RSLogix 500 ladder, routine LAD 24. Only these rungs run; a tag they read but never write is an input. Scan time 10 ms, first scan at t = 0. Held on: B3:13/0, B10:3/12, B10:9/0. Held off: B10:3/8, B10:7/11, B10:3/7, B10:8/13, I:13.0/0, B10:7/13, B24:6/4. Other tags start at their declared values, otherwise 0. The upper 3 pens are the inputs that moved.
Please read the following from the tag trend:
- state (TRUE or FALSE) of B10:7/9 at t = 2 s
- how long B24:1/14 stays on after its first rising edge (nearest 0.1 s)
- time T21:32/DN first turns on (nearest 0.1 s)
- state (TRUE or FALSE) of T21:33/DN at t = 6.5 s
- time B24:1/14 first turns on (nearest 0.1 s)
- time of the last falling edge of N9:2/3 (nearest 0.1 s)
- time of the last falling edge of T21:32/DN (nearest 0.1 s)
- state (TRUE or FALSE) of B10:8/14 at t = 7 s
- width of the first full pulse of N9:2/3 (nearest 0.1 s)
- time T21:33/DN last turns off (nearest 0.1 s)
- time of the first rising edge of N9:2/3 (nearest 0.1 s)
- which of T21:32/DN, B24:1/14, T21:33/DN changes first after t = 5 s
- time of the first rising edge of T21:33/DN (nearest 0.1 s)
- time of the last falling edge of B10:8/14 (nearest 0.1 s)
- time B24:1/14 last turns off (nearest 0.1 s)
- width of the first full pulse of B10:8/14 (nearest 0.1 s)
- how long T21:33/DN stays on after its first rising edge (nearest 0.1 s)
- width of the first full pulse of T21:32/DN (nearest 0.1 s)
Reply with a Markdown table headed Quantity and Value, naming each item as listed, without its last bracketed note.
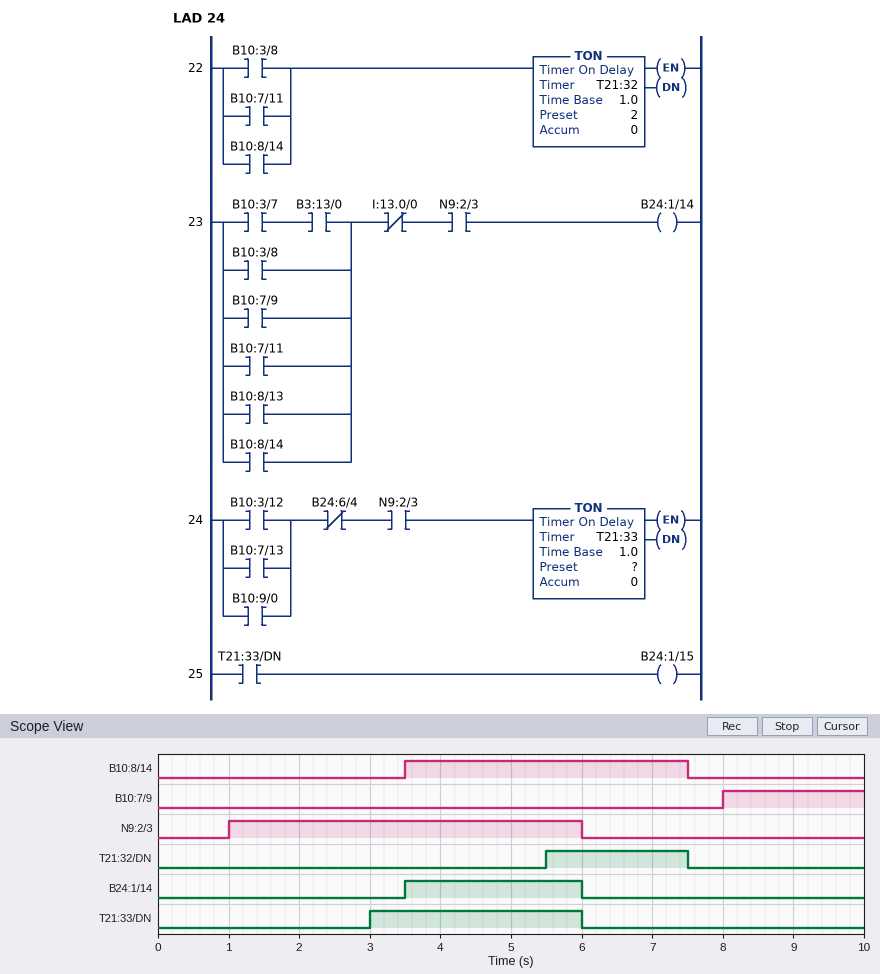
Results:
| Quantity | Value |
|---|---|
| state (TRUE or FALSE) of B10:7/9 at t = 2 s | FALSE |
| how long B24:1/14 stays on after its first rising edge | 2.5 s |
| time T21:32/DN first turns on | 5.5 s |
| state (TRUE or FALSE) of T21:33/DN at t = 6.5 s | FALSE |
| time B24:1/14 first turns on | 3.5 s |
| time of the last falling edge of N9:2/3 | 6.0 s |
| time of the last falling edge of T21:32/DN | 7.5 s |
| state (TRUE or FALSE) of B10:8/14 at t = 7 s | TRUE |
| width of the first full pulse of N9:2/3 | 5.0 s |
| time T21:33/DN last turns off | 6.0 s |
| time of the first rising edge of N9:2/3 | 1.0 s |
| which of T21:32/DN, B24:1/14, T21:33/DN changes first after t = 5 s | T21:32/DN |
| time of the first rising edge of T21:33/DN | 3.0 s |
| time of the last falling edge of B10:8/14 | 7.5 s |
| time B24:1/14 last turns off | 6.0 s |
| width of the first full pulse of B10:8/14 | 4.0 s |
| how long T21:33/DN stays on after its first rising edge | 3.0 s |
| width of the first full pulse of T21:32/DN | 2.0 s |
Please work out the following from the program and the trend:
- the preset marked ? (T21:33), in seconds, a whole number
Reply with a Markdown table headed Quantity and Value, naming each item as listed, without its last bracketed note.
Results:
| Quantity | Value |
|---|---|
| the preset marked ? (T21:33), in seconds, a whole number | 2 s |
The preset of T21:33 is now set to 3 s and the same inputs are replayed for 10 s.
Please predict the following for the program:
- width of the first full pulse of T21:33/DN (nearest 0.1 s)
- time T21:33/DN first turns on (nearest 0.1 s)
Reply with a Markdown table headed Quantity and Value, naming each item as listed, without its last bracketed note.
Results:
| Quantity | Value |
|---|---|
| width of the first full pulse of T21:33/DN | 2.0 s |
| time T21:33/DN first turns on | 4.0 s |
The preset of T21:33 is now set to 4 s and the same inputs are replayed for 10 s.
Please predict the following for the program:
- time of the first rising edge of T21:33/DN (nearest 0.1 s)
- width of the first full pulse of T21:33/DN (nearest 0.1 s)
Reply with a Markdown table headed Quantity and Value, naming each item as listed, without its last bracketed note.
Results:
| Quantity | Value |
|---|---|
| time of the first rising edge of T21:33/DN | 5.0 s |
| width of the first full pulse of T21:33/DN | 1.0 s |
